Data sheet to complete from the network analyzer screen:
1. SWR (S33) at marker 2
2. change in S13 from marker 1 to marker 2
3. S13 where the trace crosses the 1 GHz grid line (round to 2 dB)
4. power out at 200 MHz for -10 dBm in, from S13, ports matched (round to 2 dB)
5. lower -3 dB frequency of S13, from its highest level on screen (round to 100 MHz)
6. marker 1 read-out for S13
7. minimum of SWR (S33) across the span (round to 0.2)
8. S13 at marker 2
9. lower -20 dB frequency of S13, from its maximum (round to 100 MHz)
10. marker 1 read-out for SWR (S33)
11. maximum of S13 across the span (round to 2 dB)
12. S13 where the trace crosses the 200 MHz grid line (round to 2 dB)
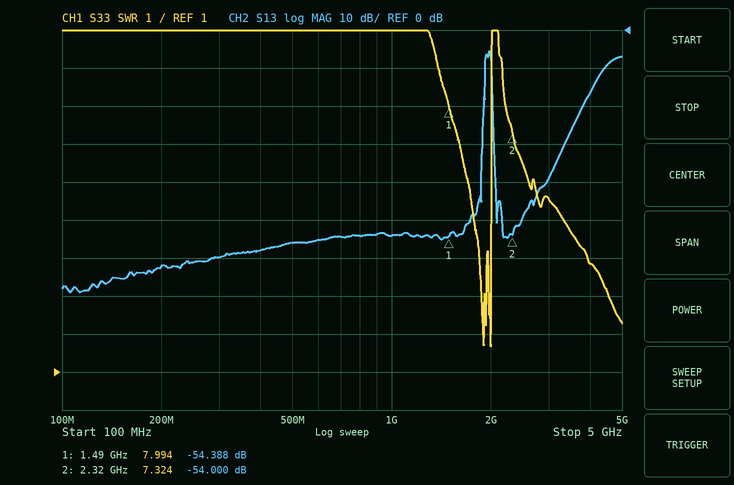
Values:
7.324
0.388 dB
-54 dB
-72 dBm
1.9 GHz
-54.388 dB
1.6
-54.000 dB
1.9 GHz
7.994
-6 dB
-62 dB
